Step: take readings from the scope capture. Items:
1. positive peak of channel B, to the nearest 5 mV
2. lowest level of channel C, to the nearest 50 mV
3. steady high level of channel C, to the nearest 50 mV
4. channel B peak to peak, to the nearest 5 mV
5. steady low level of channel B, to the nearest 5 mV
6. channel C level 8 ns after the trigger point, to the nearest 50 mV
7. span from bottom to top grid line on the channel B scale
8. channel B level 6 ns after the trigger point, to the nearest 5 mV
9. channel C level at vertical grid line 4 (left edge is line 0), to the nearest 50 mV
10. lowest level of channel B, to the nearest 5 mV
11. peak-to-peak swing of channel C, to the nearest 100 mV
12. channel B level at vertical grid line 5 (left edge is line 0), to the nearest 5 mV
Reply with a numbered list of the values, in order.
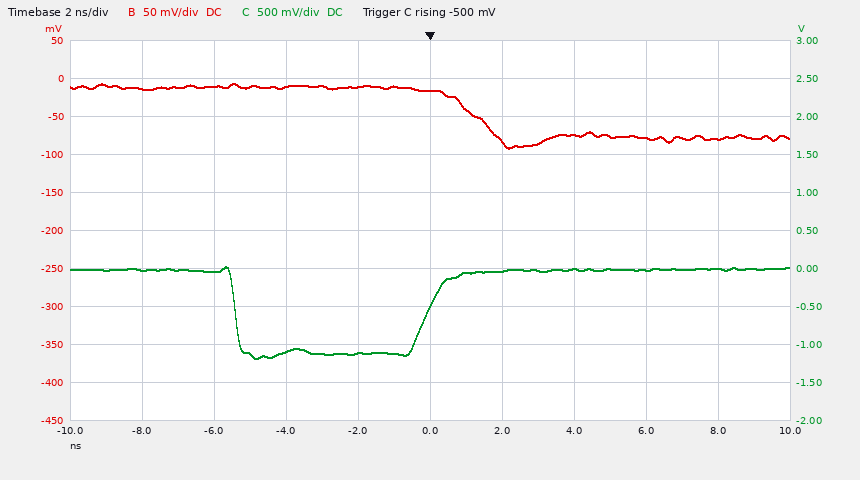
1. -5 mV
2. -1.20 V
3. 0 mV
4. 85 mV
5. -75 mV
6. 0 mV
7. 500 mV
8. -80 mV
9. -1.10 V
10. -90 mV
11. 1.20 V
12. -15 mV
